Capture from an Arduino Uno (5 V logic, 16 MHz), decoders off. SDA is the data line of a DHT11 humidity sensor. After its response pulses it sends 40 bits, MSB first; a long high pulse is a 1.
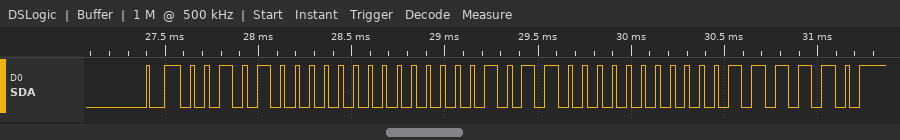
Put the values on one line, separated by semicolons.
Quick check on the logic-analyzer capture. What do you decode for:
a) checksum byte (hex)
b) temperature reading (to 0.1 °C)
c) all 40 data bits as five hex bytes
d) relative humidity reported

0x3E; 22.0 °C; 28 00 16 00 3E; 40 %
